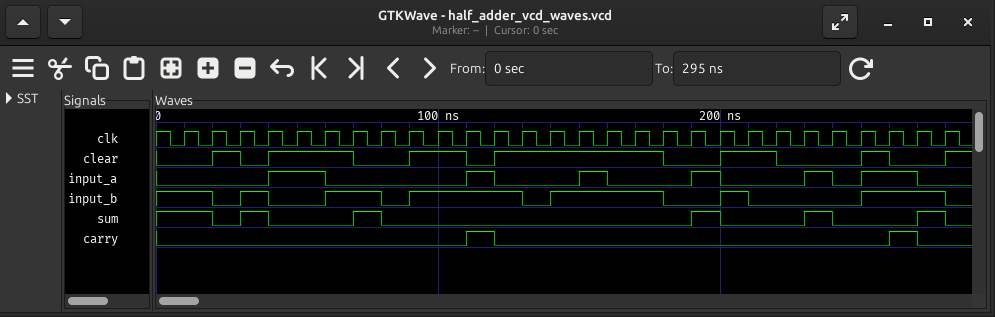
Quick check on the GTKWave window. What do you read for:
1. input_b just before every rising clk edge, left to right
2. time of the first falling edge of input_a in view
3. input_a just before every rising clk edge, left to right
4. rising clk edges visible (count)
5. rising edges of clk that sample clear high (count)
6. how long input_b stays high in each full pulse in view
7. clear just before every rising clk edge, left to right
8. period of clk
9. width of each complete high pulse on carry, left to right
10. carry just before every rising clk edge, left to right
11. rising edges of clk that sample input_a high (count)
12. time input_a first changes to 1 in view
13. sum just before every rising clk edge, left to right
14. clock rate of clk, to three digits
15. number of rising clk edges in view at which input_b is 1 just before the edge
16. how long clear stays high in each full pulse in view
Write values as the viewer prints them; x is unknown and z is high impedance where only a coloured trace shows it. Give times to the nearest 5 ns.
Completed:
1 1 0 1 0 0 1 1 0 1 1 1 1 0 1 1 1 1 0 0 1 0 0 0 0 1 1 1
60 ns
0 0 0 0 1 1 0 0 0 0 0 1 0 0 0 1 0 0 0 1 0 0 0 1 0 1 1 0
28
15
10 ns, 20 ns, 40 ns, 40 ns, 10 ns, 30 ns
0 0 1 0 1 1 1 0 0 1 1 0 1 1 1 1 1 1 0 0 1 1 0 0 0 1 0 0
10 ns
10 ns, 10 ns
0 0 0 0 0 0 0 0 0 0 0 1 0 0 0 0 0 0 0 0 0 0 0 0 0 0 1 0
8
40 ns
1 1 0 1 0 0 0 1 0 0 0 0 0 0 0 0 0 0 0 1 0 0 0 1 0 0 0 1
100 MHz
17
10 ns, 30 ns, 20 ns, 60 ns, 20 ns, 10 ns
